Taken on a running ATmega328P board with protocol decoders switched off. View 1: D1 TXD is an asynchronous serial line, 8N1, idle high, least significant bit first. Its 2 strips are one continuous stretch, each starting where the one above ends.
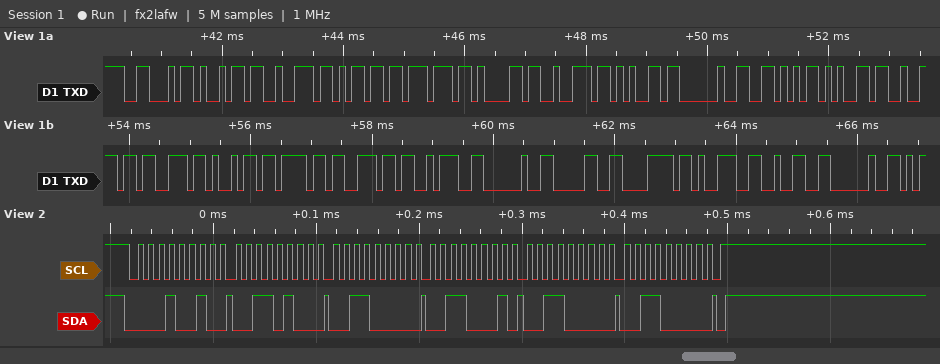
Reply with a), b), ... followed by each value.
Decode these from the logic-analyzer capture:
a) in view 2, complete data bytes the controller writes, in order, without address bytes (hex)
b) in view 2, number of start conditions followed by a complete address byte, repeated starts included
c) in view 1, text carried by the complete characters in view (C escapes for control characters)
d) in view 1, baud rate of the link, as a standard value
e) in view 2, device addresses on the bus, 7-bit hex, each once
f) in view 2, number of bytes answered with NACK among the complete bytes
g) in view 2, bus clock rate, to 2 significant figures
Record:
a) 34 30 31 30 30
b) 1
c) "Firmware Version: 0x92 "
d) 9600 baud
e) 0x09
f) 0
g) 100 kHz
